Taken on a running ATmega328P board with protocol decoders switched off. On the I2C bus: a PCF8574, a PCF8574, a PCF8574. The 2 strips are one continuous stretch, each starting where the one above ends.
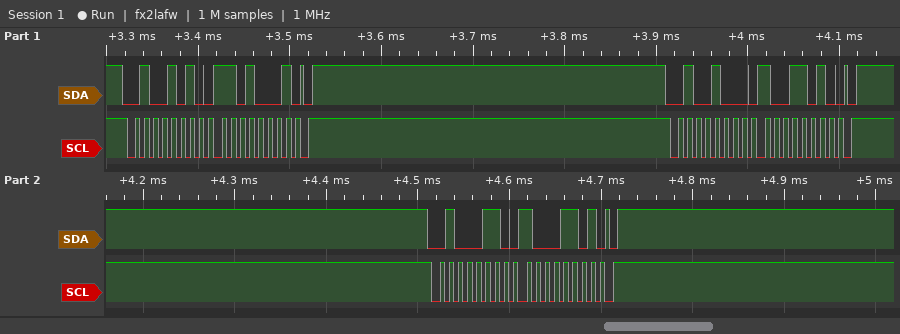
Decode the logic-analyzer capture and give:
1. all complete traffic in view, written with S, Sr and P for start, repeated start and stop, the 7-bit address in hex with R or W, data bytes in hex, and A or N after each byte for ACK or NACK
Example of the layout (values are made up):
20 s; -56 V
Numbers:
S 25W A D1 A P S 24W A 9A A P S 23W A 8D A P
